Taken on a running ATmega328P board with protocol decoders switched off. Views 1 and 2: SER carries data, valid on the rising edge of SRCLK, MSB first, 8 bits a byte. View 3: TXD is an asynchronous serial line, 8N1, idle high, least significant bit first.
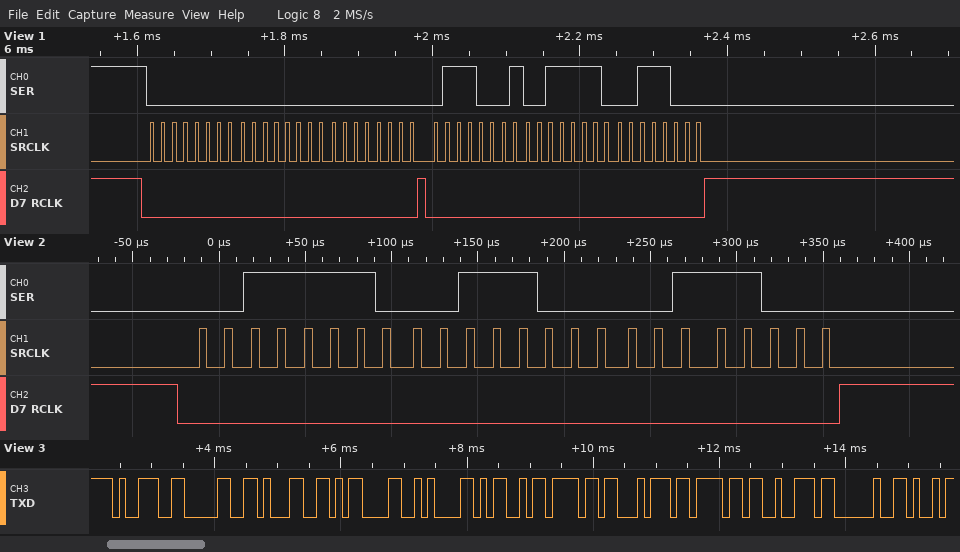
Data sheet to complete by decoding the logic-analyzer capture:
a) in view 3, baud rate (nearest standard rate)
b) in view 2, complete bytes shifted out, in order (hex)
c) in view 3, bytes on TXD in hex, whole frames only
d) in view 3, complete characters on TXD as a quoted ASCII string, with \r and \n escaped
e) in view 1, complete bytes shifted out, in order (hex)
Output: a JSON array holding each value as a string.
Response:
["9600 baud", "3E 38 38", "0x39 0x30 0x31 0x0D 0x0A 0x4D 0x6F 0x74 0x6F 0x72 0x20", "\"901\\r\\nMotor \"", "00 00 00 71 3E 38"]
